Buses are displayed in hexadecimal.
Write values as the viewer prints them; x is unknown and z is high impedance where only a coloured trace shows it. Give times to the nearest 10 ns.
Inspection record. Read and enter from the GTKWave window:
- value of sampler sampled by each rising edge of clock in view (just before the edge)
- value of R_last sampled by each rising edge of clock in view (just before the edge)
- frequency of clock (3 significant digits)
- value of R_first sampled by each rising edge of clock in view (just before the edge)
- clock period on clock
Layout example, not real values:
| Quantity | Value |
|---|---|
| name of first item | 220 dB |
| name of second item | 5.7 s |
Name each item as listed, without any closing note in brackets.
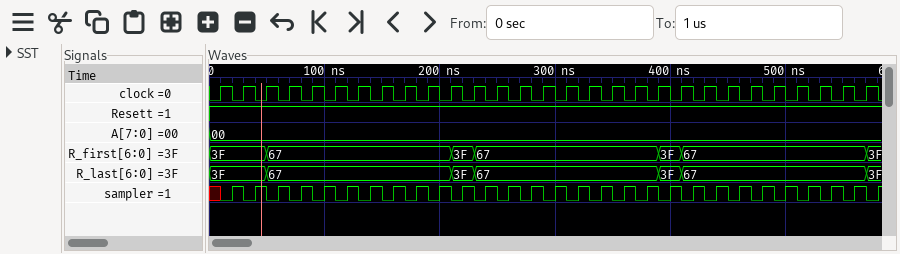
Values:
| Quantity | Value |
|---|---|
| value of sampler sampled by each rising edge of clock in view | x 1 1 1 1 1 1 1 1 1 1 1 1 1 1 1 1 1 1 1 1 1 1 1 1 1 1 1 1 |
| value of R_last sampled by each rising edge of clock in view | 3F, 3F, 3F, 67, 67, 67, 67, 67, 67, 67, 67, 3F, 67, 67, 67, 67, 67, 67, 67, 67, 3F, 67, 67, 67, 67, 67, 67, 67, 67 |
| frequency of clock | 50.0 MHz |
| value of R_first sampled by each rising edge of clock in view | 3F, 3F, 3F, 67, 67, 67, 67, 67, 67, 67, 67, 3F, 67, 67, 67, 67, 67, 67, 67, 67, 3F, 67, 67, 67, 67, 67, 67, 67, 67 |
| clock period on clock | 20 ns |
